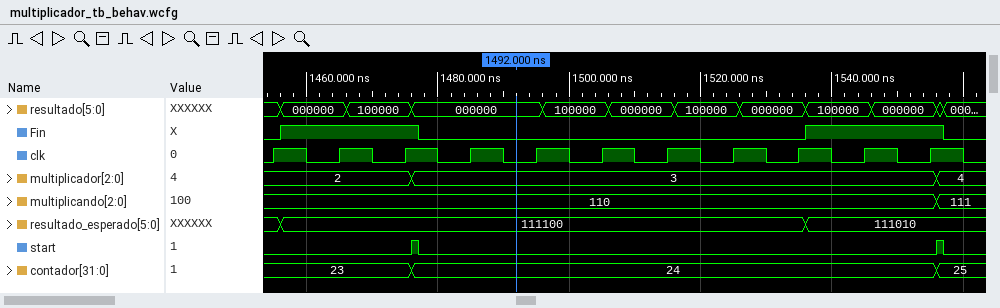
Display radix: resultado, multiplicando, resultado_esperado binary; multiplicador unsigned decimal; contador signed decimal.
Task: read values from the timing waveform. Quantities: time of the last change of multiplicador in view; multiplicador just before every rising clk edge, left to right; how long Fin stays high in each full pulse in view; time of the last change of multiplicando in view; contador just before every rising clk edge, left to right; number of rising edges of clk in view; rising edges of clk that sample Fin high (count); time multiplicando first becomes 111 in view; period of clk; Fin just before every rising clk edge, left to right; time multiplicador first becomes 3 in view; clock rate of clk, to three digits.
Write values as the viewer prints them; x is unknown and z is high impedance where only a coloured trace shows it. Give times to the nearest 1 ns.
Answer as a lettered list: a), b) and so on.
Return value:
a) 1556 ns
b) 2, 2, 2, 3, 3, 3, 3, 3, 3, 3, 3
c) 21 ns, 21 ns
d) 1556 ns
e) 23, 23, 23, 24, 24, 24, 24, 24, 24, 24, 24
f) 11
g) 4
h) 1556 ns
i) 10 ns
j) 0 1 1 0 0 0 0 0 0 1 1
k) 1476 ns
l) 100 MHz
